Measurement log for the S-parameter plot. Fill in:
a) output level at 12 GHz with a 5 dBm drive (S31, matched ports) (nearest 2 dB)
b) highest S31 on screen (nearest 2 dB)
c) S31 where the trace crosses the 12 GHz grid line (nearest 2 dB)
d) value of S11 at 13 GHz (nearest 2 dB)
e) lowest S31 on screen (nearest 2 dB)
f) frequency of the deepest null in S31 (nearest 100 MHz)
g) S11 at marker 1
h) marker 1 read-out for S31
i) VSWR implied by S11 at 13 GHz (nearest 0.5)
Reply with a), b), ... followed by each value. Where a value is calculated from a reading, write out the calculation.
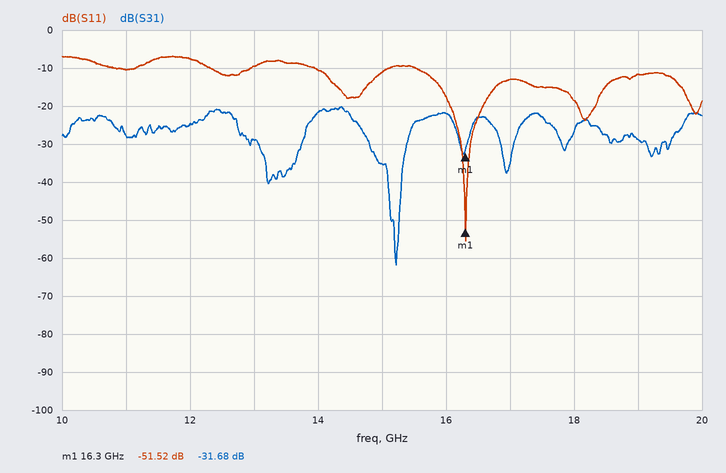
a) 5 dBm + (-24 dB) = -20 dBm
b) -20 dB
c) -24 dB
d) -10 dB
e) -62 dB
f) 15.2 GHz
g) -51.52 dB
h) -31.68 dB
i) |Γ| = 10^(-10/20) = 0.3162; VSWR = (1 + 0.3162)/(1 − 0.3162) ≈ 1.92, so 2.0 to the nearest 0.5
